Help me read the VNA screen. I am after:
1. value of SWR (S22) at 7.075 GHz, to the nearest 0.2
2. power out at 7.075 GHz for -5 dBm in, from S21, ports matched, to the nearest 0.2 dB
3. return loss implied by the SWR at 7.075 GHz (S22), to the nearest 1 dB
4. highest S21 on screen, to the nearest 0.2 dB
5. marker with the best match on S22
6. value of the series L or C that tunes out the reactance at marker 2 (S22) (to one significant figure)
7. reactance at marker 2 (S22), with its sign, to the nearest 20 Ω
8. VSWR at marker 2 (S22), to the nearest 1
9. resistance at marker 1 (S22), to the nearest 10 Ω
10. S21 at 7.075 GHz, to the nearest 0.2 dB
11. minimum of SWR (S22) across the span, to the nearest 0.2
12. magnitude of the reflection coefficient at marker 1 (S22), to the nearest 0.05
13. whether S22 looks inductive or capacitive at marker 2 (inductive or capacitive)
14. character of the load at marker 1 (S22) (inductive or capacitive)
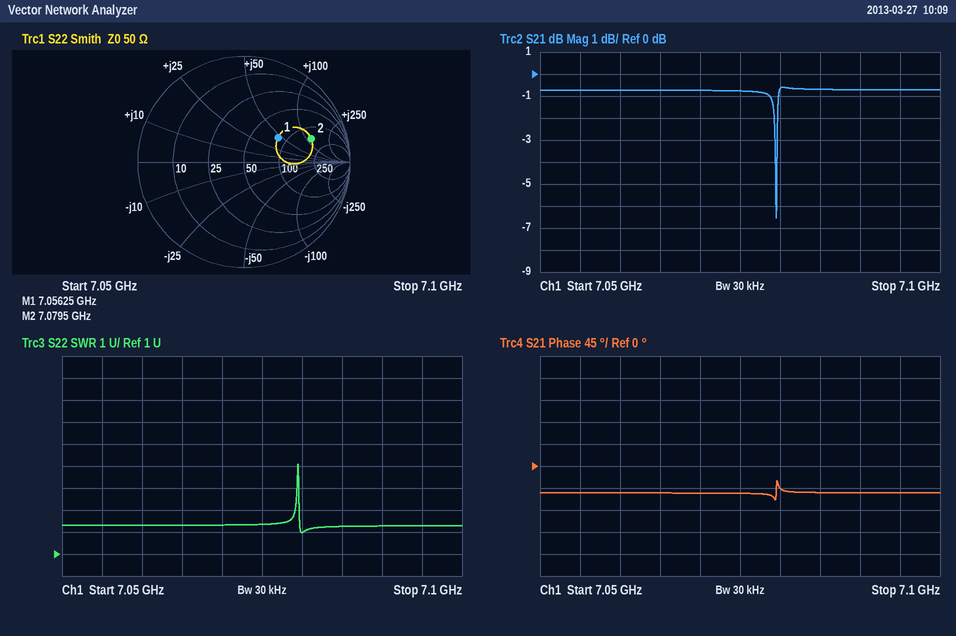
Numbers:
2.4
-5.8 dBm
8 dB
-0.6 dB
marker 1
200 fF
+120 Ω
5
80 Ω
-0.8 dB
2.0
0.40
inductive
inductive
